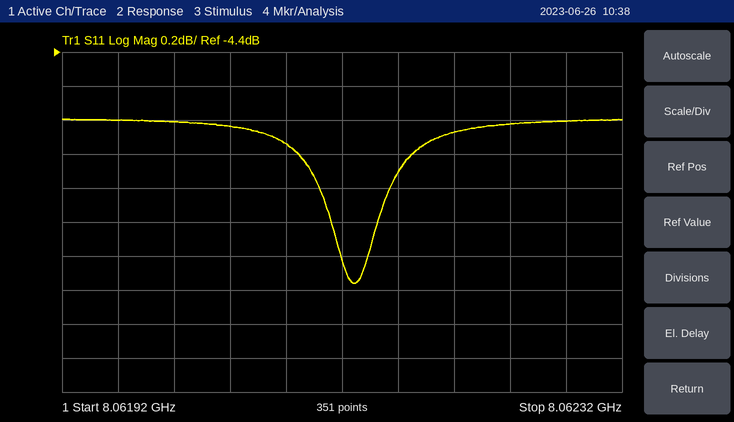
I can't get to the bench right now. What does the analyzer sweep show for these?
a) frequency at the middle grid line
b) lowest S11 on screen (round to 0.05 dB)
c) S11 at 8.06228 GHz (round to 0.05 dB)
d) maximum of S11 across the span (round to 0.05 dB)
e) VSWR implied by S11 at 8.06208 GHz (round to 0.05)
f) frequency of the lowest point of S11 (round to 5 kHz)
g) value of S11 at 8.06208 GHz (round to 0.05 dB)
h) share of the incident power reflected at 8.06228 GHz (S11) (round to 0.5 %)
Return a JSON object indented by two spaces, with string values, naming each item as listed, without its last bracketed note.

{
  "frequency at the middle grid line": "8.06212 GHz",
  "lowest S11 on screen": "-5.75 dB",
  "S11 at 8.06228 GHz": "-4.80 dB",
  "maximum of S11 across the span": "-4.80 dB",
  "VSWR implied by S11 at 8.06208 GHz": "3.60",
  "frequency of the lowest point of S11": "8.062130 GHz",
  "value of S11 at 8.06208 GHz": "-4.95 dB",
  "share of the incident power reflected at 8.06228 GHz (S11)": "33.0 %"
}
